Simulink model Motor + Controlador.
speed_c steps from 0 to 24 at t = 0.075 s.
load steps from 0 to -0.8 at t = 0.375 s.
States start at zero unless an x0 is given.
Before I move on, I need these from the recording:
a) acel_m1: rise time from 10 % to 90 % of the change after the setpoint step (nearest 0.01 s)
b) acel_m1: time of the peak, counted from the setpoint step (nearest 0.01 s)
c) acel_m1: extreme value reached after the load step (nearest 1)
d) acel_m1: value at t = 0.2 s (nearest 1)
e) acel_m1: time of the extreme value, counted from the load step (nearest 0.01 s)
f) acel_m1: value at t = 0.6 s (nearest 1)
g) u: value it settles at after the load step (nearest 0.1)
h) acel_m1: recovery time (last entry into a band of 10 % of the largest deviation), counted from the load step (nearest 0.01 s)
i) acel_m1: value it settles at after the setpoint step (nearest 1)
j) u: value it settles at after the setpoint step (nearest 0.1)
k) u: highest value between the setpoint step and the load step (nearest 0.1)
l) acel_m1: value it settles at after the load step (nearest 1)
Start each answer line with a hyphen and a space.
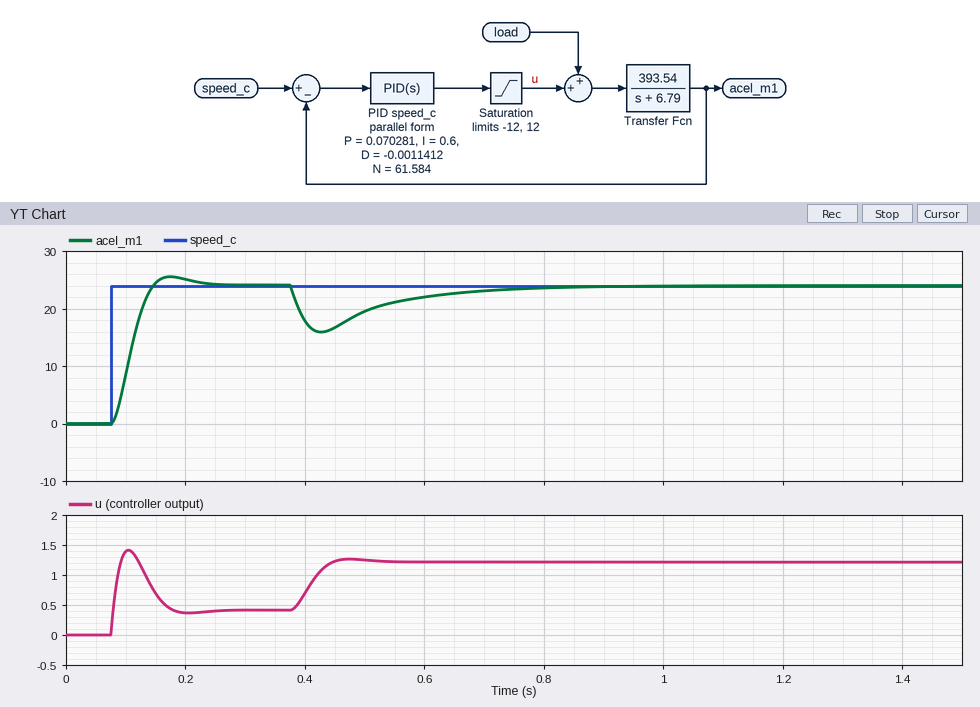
- 0.05 s
- 0.10 s
- 16
- 25
- 0.05 s
- 22
- 1.2
- 0.34 s
- 24
- 0.4
- 1.4
- 24
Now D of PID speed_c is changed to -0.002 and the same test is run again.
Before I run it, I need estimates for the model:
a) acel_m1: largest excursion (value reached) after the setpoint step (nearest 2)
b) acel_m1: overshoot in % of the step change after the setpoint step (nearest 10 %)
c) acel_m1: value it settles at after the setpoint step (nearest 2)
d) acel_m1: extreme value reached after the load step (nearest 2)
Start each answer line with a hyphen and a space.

- 30
- 20 %
- 24
- 14
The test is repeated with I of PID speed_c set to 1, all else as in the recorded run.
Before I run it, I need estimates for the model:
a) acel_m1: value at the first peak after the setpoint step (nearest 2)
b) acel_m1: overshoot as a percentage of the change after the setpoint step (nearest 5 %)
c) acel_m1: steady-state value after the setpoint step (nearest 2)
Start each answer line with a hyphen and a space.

- 28
- 15 %
- 24
